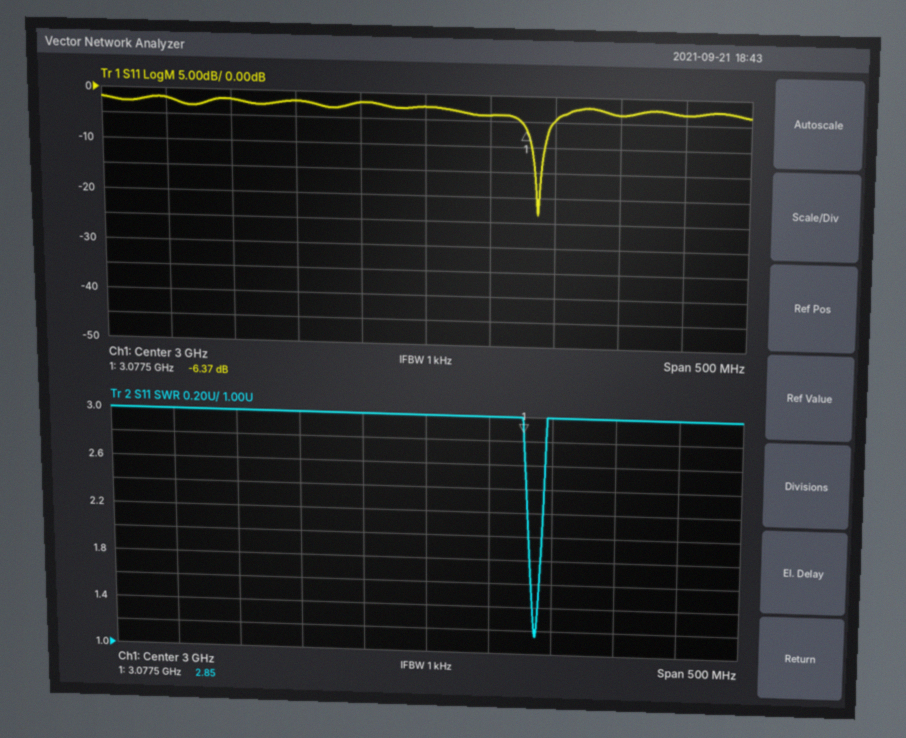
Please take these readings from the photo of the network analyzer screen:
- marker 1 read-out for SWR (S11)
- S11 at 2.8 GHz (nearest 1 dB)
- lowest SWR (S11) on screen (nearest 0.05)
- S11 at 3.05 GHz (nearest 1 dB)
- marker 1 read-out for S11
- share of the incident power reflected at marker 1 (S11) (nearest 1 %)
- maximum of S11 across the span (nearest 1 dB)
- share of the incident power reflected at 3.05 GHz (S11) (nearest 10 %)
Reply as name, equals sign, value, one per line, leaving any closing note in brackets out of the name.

marker 1 read-out for SWR = 2.85
S11 at 2.8 GHz = -2 dB
lowest SWR (S11) on screen = 1.15
S11 at 3.05 GHz = -4 dB
marker 1 read-out for S11 = -6.37 dB
share of the incident power reflected at marker 1 (S11) = 23 %
maximum of S11 across the span = -2 dB
share of the incident power reflected at 3.05 GHz (S11) = 40 %
